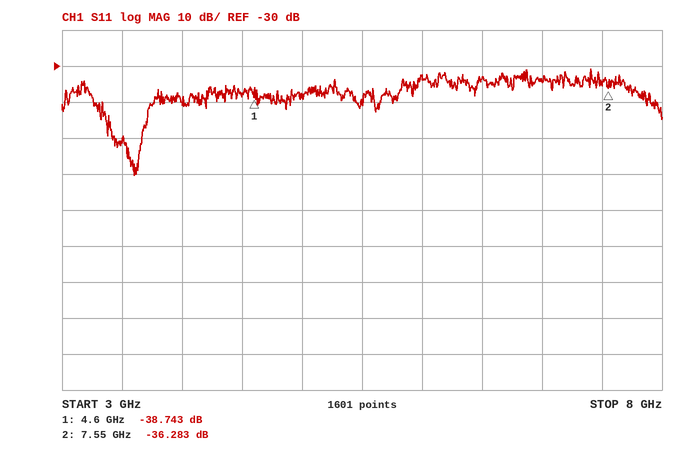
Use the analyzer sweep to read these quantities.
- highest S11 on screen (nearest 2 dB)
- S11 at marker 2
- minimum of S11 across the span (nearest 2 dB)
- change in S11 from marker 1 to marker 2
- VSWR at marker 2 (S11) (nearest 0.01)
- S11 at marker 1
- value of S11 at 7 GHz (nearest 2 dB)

-30 dB
-36.283 dB
-60 dB
2.460 dB
1.03
-38.743 dB
-34 dB
